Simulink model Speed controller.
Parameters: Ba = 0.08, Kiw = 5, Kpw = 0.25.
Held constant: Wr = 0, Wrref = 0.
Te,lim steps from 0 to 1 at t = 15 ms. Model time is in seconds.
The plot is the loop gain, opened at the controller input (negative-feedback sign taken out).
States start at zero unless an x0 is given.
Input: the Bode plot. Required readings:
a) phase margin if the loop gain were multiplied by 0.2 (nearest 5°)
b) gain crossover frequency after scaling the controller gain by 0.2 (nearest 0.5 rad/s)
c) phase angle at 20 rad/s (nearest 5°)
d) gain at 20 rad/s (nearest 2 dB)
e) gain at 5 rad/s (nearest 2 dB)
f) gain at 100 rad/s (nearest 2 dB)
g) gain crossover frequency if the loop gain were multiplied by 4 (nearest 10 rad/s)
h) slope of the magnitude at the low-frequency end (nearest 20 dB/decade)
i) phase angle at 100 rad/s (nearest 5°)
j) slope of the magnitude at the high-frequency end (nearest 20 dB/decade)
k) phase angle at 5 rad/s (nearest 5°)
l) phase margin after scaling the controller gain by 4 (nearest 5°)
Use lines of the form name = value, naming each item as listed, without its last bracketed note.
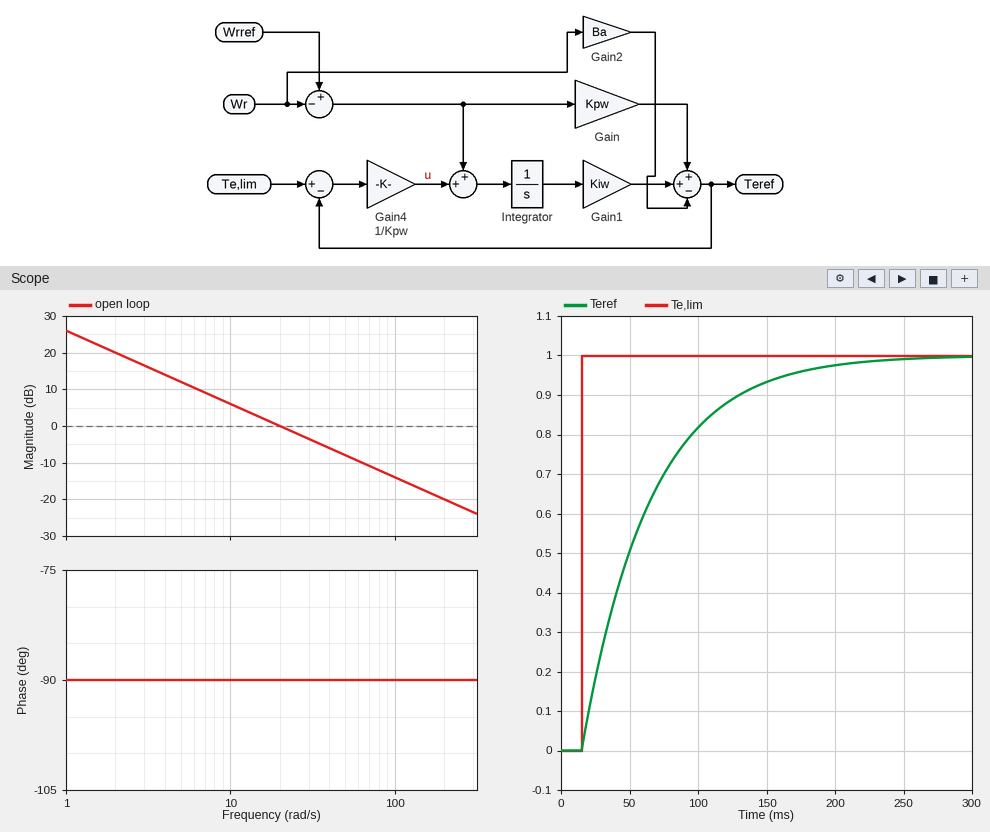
phase margin if the loop gain were multiplied by 0.2 = 90°
gain crossover frequency after scaling the controller gain by 0.2 = 4.0 rad/s
phase angle at 20 rad/s = -90°
gain at 20 rad/s = 0 dB
gain at 5 rad/s = 12 dB
gain at 100 rad/s = -14 dB
gain crossover frequency if the loop gain were multiplied by 4 = 80 rad/s
slope of the magnitude at the low-frequency end = -20 dB/decade
phase angle at 100 rad/s = -90°
slope of the magnitude at the high-frequency end = -20 dB/decade
phase angle at 5 rad/s = -90°
phase margin after scaling the controller gain by 4 = 90°
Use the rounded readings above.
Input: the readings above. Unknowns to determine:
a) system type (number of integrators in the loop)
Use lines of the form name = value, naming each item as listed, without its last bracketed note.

system type = 1
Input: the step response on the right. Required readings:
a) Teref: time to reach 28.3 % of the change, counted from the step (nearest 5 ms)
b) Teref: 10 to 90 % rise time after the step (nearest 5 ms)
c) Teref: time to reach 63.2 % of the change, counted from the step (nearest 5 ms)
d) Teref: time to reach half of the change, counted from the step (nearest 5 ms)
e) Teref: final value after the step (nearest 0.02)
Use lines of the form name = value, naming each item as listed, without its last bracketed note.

Teref: time to reach 28.3 % of the change, counted from the step = 15 ms
Teref: 10 to 90 % rise time after the step = 110 ms
Teref: time to reach 63.2 % of the change, counted from the step = 50 ms
Teref: time to reach half of the change, counted from the step = 35 ms
Teref: final value after the step = 1.00
